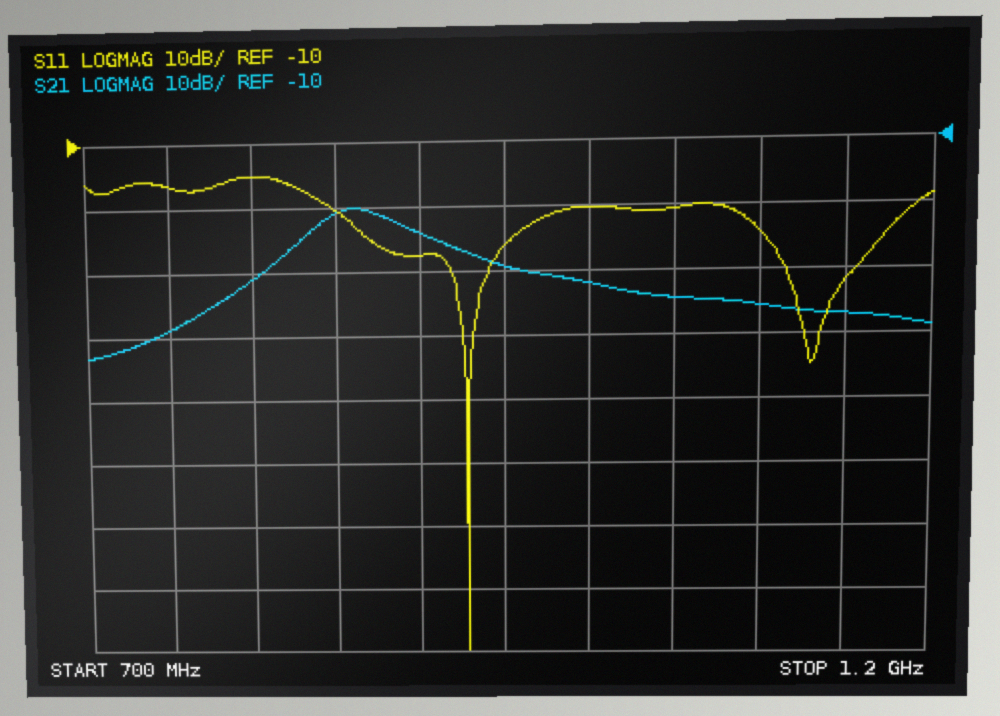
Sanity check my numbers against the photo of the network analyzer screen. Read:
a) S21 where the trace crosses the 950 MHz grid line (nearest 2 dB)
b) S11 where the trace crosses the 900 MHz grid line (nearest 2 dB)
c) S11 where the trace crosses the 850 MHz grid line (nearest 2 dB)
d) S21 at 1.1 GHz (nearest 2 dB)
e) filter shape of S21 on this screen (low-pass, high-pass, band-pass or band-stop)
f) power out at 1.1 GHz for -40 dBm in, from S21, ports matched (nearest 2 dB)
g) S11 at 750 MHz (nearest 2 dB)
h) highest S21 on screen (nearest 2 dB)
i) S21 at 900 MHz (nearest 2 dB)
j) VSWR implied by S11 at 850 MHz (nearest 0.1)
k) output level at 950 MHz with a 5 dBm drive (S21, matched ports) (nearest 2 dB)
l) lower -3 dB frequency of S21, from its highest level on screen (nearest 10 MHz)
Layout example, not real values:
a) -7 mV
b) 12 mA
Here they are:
a) -30 dB
b) -28 dB
c) -20 dB
d) -36 dB
e) band-pass
f) -76 dBm
g) -16 dB
h) -20 dB
i) -24 dB
j) 1.2
k) -24 dBm
l) 840 MHz
